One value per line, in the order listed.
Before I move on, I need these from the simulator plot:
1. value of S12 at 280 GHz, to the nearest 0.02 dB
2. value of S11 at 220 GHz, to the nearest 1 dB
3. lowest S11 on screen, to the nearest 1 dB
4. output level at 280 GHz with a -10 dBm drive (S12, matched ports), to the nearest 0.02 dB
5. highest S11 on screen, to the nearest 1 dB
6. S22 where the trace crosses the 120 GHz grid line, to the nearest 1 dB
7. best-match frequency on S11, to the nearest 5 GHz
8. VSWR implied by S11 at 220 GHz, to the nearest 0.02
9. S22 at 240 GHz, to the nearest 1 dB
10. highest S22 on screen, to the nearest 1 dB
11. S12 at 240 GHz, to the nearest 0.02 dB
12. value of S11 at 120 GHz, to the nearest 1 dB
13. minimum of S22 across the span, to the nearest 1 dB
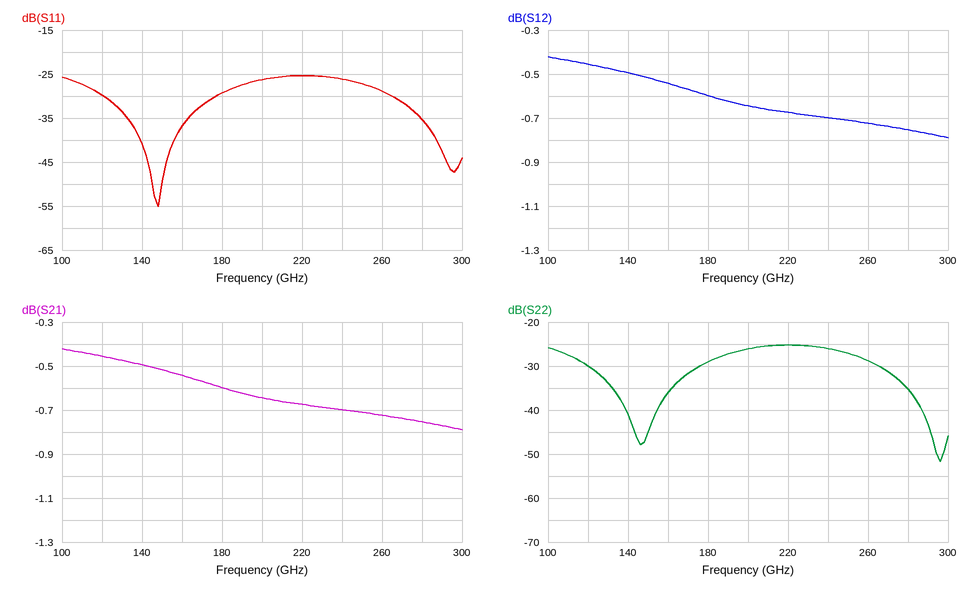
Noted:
-0.76 dB
-25 dB
-55 dB
-10.76 dBm
-25 dB
-30 dB
150 GHz
1.12
-26 dB
-25 dB
-0.70 dB
-30 dB
-52 dB
